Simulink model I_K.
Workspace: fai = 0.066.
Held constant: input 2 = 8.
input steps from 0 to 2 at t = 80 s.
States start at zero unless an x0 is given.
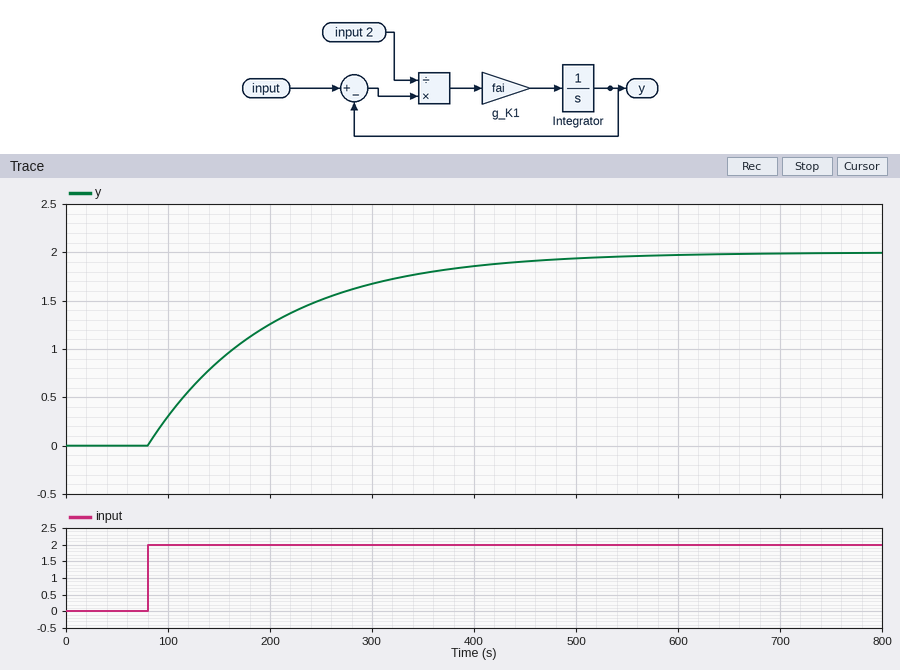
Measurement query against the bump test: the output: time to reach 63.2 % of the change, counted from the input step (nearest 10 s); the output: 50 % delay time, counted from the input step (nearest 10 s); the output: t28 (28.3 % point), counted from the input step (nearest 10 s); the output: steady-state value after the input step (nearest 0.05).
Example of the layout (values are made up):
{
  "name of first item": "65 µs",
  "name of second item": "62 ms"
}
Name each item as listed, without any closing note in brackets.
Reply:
{
  "the output: time to reach 63.2 % of the change, counted from the input step": "120 s",
  "the output: 50 % delay time, counted from the input step": "80 s",
  "the output: t28 (28.3 % point), counted from the input step": "40 s",
  "the output: steady-state value after the input step": "2.00"
}
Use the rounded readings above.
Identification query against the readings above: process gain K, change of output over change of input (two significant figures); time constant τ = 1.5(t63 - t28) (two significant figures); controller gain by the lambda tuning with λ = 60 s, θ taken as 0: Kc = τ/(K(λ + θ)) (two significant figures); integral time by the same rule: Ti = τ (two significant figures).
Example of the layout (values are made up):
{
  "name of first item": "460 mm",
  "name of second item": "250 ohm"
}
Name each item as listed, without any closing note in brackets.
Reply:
{
  "process gain K, change of output over change of input": "1.0",
  "time constant τ = 1.5(t63 - t28)": "120 s",
  "controller gain by the lambda tuning with λ = 60 s, θ taken as 0: Kc = τ/(K(λ + θ))": "2.0",
  "integral time by the same rule: Ti = τ": "120 s"
}
